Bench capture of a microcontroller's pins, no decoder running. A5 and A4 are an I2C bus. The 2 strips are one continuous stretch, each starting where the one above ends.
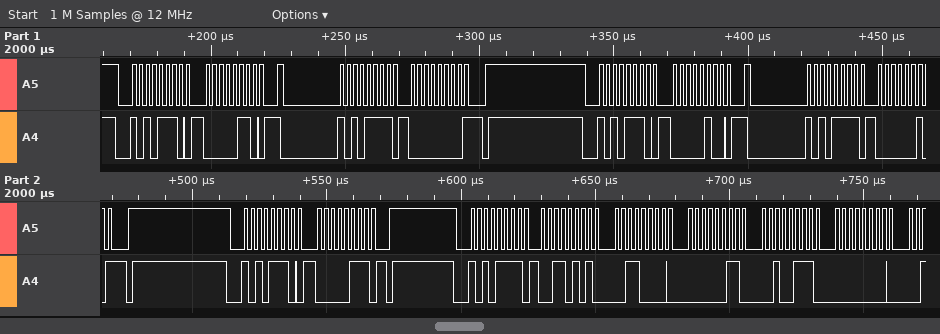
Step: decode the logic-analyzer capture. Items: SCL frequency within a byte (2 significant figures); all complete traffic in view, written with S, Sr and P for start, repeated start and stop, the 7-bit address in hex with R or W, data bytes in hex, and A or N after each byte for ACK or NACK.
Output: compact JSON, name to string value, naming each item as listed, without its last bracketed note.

{"SCL frequency within a byte": "400 kHz", "all complete traffic in view, written with S, Sr and P for start, repeated start and stop, the 7-bit address in hex with R or W, data bytes in hex, and A or N after each byte for ACK or NACK": "S 57W A 06 A Sr 57R A 00 N P S 57W A 04 A Sr 57R A 02 N P S 57W A 07 A P S 57R A 35 A 30 A 03 A 27 A 00 A"}
